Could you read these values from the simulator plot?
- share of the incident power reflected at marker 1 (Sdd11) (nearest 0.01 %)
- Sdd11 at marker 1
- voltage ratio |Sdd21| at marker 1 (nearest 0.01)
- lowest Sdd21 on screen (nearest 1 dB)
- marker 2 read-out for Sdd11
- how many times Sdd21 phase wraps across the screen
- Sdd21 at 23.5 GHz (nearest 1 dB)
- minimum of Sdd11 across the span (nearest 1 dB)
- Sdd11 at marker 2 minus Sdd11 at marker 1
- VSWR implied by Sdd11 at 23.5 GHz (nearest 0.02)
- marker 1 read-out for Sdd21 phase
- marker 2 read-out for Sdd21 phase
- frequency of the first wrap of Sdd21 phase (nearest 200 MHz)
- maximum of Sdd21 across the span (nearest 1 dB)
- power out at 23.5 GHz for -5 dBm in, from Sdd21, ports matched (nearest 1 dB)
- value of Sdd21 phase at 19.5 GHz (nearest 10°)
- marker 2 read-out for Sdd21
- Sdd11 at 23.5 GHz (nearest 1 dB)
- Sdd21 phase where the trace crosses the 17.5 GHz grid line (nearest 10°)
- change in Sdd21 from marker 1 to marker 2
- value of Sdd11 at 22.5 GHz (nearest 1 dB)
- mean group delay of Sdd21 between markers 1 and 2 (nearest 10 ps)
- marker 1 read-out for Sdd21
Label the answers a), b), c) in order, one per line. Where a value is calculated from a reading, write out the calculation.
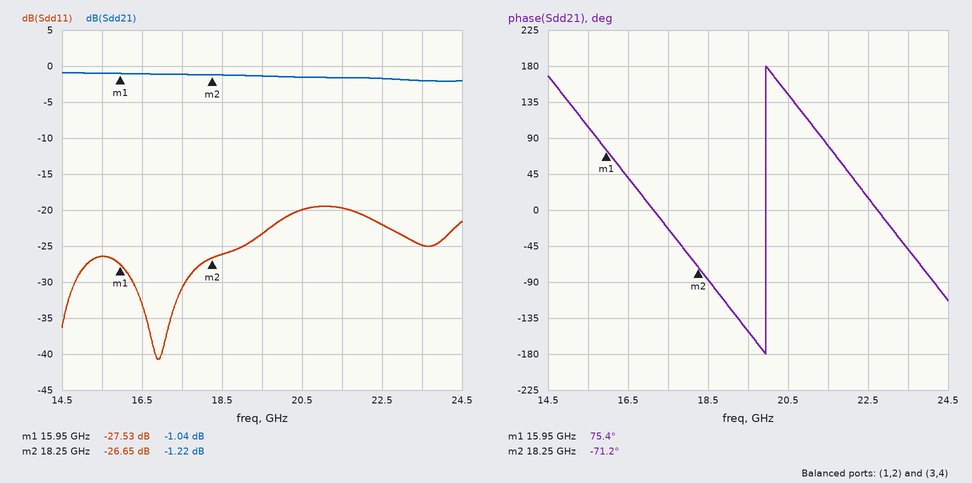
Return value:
a) 10^(-27.53/10) ≈ 0.18 %
b) -27.53 dB
c) 10^(-1.04/20) ≈ 0.89
d) -2 dB
e) -26.65 dB
f) 1
g) -2 dB
h) -41 dB
i) -26.65 − (-27.53) = 0.88 dB
j) |Γ| = 10^(-25/20) = 0.0562; VSWR = (1 + 0.0562)/(1 − 0.0562) ≈ 1.12
k) 75.4°
l) -71.2°
m) 20.0 GHz
n) -1 dB
o) -5 dBm + (-2 dB) = -7 dBm
p) -150°
q) -1.22 dB
r) -25 dB
s) -20°
t) -1.22 − (-1.04) = -0.18 dB
u) -22 dB
v) −(-71.2° − (75.4°))/(360° × 2.3 GHz) ≈ 177 ps, so 180 ps to the nearest 10 ps
w) -1.04 dB
